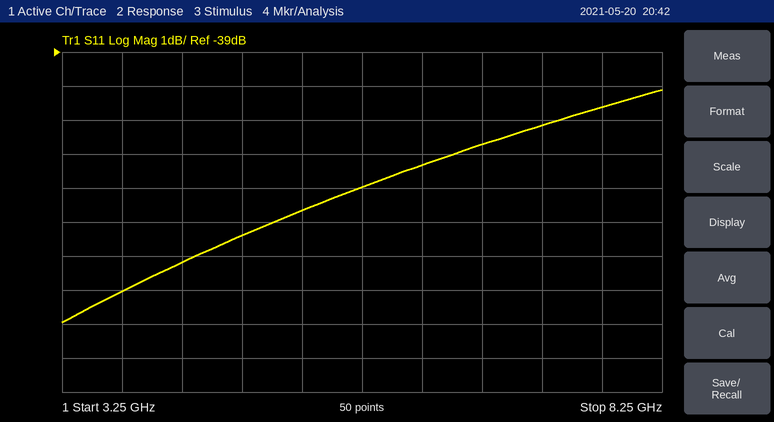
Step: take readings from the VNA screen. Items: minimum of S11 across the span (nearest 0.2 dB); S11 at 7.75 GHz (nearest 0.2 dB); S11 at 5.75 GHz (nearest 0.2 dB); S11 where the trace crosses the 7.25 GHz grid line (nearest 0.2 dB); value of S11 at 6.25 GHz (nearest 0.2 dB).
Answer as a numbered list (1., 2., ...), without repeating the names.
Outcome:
1. -47.0 dB
2. -40.6 dB
3. -43.0 dB
4. -41.2 dB
5. -42.4 dB
